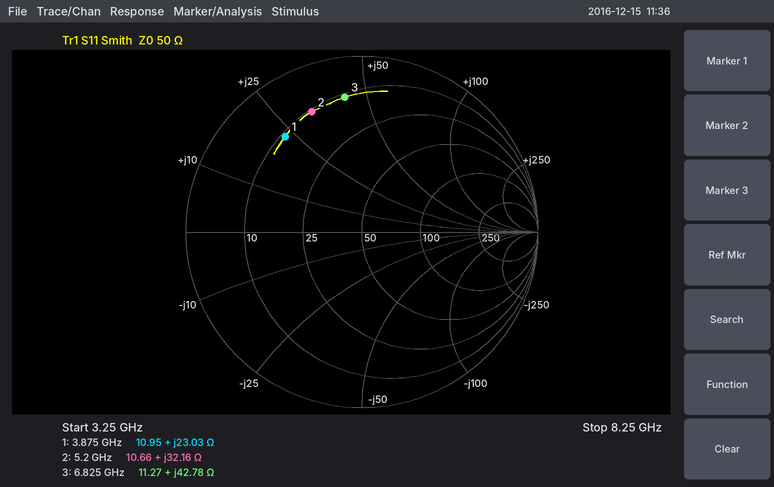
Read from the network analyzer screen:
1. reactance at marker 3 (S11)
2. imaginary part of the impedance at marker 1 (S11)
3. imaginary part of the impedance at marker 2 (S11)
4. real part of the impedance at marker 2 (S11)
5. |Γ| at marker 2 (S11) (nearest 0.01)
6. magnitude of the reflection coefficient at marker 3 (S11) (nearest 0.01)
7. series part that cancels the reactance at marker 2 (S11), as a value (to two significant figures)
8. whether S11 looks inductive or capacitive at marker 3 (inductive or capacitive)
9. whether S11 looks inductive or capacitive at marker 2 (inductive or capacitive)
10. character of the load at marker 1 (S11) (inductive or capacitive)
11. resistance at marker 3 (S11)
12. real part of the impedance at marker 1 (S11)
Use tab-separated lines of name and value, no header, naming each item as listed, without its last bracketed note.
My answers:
reactance at marker 3	+42.78 Ω
imaginary part of the impedance at marker 1	+23.03 Ω
imaginary part of the impedance at marker 2	+32.16 Ω
real part of the impedance at marker 2	10.66 Ω
|Γ| at marker 2 (S11)	0.74
magnitude of the reflection coefficient at marker 3 (S11)	0.77
series part that cancels the reactance at marker 2 (S11), as a value	950 fF
whether S11 looks inductive or capacitive at marker 3	inductive
whether S11 looks inductive or capacitive at marker 2	inductive
character of the load at marker 1 (S11)	inductive
resistance at marker 3	11.27 Ω
real part of the impedance at marker 1	10.95 Ω
